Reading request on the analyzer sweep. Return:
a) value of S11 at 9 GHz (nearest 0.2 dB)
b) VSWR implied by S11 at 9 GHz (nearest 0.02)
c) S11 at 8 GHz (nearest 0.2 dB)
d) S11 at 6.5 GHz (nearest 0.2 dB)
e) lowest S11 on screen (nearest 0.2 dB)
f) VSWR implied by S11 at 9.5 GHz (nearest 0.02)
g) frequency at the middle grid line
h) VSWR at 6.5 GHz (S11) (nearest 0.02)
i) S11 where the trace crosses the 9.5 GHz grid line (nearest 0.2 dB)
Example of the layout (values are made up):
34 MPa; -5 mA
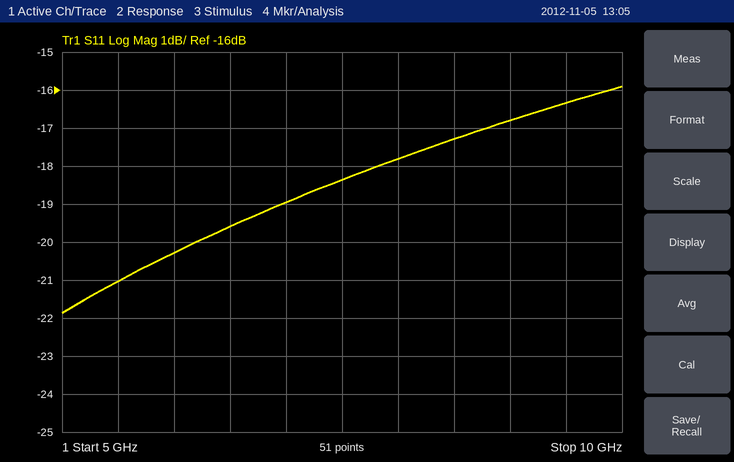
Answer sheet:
-16.8 dB; 1.34; -17.8 dB; -19.6 dB; -21.8 dB; 1.36; 7.5 GHz; 1.24; -16.4 dB
